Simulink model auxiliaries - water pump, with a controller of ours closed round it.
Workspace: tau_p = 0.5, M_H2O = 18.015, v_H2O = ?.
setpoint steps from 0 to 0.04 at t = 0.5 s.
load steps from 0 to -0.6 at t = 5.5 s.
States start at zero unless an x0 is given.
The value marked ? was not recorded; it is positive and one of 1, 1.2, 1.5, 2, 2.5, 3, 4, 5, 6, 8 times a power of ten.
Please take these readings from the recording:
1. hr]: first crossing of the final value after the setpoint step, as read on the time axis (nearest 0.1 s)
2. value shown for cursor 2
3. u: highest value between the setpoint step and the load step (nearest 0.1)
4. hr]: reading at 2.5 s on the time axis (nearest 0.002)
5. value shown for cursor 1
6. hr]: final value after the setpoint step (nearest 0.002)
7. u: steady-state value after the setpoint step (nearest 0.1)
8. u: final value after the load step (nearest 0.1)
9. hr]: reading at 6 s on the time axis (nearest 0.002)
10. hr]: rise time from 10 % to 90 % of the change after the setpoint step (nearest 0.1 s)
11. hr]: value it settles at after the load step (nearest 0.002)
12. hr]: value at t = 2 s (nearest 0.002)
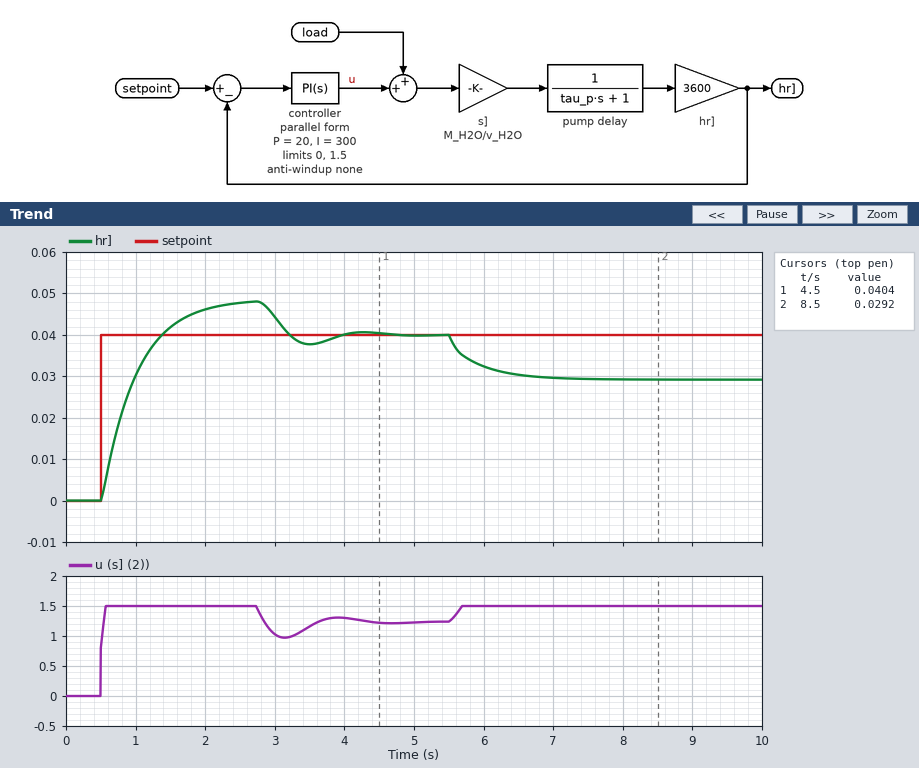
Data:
1.4 s
0.0292
1.5
0.048
0.0404
0.040
1.2
1.5
0.032
0.6 s
0.030
0.046
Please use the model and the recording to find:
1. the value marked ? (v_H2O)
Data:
2e+06
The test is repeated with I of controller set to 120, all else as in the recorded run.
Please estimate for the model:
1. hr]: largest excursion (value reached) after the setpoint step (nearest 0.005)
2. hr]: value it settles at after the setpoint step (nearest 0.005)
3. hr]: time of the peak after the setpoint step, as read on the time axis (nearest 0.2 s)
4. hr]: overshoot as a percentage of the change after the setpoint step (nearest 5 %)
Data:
0.045
0.040
2.0 s
15 %
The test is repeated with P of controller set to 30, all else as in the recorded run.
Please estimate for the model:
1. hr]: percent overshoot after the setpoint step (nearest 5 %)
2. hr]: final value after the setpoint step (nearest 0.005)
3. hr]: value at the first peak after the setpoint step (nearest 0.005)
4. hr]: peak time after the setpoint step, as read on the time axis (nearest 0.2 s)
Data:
20 %
0.040
0.050
2.6 s
